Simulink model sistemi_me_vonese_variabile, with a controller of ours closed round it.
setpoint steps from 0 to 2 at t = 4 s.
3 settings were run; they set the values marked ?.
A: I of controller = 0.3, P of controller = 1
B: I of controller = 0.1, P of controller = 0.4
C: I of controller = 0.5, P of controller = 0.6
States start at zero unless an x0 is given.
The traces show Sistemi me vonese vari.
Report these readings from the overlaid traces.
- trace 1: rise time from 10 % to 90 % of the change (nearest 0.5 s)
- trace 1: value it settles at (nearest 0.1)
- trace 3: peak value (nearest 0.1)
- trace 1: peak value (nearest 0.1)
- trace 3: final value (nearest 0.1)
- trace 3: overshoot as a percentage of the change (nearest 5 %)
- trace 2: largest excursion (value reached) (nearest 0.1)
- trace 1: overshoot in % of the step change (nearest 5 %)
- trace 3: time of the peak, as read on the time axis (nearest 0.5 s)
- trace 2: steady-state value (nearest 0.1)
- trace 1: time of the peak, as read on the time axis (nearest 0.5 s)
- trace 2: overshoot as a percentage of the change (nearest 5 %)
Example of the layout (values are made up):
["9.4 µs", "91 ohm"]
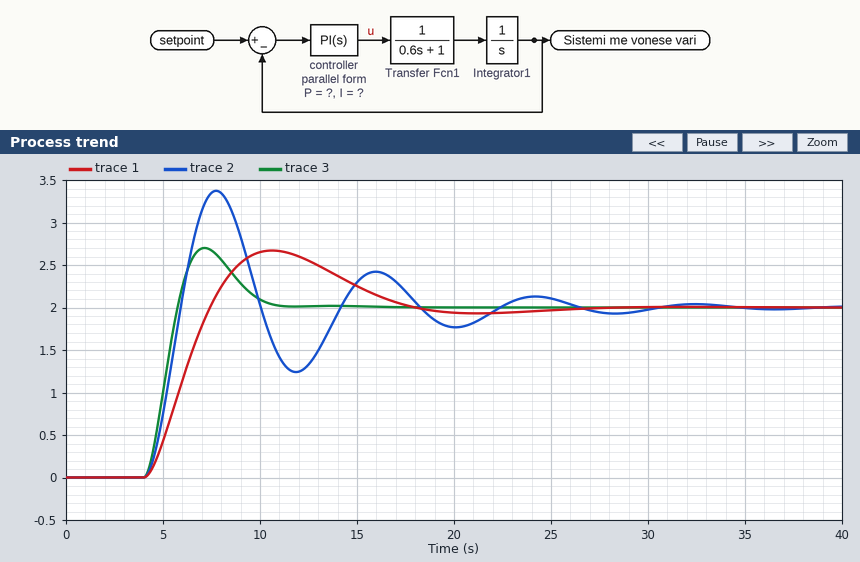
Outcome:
["2.5 s", "2.0", "2.7", "2.7", "2.0", "35 %", "3.4", "35 %", "7.0 s", "2.0", "10.5 s", "70 %"]
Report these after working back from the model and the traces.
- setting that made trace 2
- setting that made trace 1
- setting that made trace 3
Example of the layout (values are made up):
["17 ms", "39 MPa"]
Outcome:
["C", "B", "A"]
